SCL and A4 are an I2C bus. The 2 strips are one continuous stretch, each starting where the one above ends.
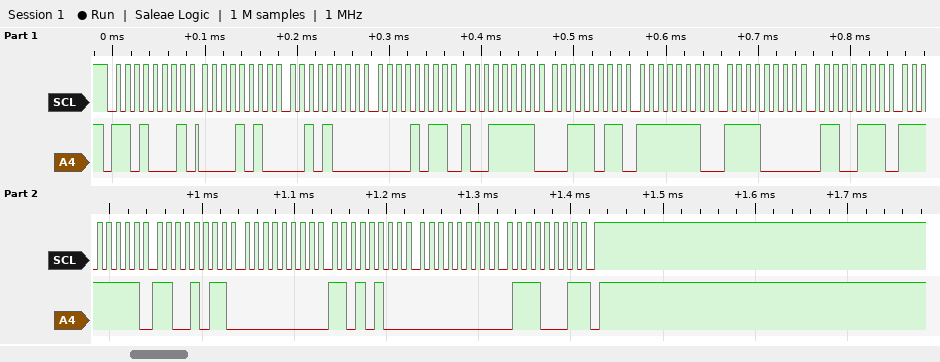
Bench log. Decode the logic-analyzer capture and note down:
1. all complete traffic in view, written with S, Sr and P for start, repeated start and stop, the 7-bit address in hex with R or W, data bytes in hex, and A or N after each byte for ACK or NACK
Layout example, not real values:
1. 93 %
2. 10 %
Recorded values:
1. S 68R A 0A A 28 A 0B A 9F A 3B A FE A F0 A 67 A FF A CB A 00 A D4 A 00 A 71 N P
